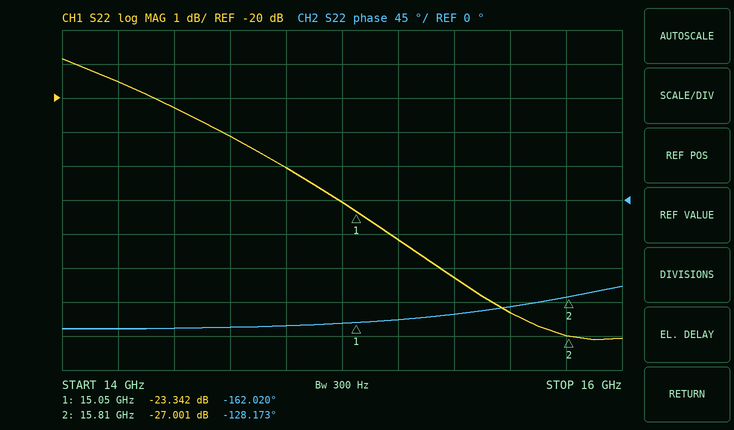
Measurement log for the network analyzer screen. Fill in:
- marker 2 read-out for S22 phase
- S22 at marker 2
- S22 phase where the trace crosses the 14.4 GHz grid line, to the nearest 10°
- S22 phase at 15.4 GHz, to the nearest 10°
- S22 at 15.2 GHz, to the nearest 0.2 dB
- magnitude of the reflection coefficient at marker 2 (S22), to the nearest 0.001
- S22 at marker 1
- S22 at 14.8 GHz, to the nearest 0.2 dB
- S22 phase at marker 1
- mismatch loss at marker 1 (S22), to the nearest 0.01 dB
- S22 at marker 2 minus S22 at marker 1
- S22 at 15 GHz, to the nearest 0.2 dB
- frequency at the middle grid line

-128.173°
-27.001 dB
-170°
-150°
-24.2 dB
0.045
-23.342 dB
-22.0 dB
-162.020°
0.02 dB
-3.659 dB
-23.0 dB
15 GHz
